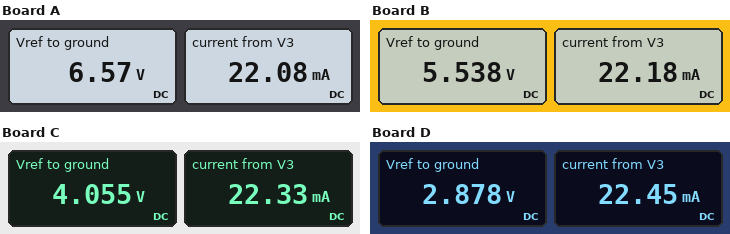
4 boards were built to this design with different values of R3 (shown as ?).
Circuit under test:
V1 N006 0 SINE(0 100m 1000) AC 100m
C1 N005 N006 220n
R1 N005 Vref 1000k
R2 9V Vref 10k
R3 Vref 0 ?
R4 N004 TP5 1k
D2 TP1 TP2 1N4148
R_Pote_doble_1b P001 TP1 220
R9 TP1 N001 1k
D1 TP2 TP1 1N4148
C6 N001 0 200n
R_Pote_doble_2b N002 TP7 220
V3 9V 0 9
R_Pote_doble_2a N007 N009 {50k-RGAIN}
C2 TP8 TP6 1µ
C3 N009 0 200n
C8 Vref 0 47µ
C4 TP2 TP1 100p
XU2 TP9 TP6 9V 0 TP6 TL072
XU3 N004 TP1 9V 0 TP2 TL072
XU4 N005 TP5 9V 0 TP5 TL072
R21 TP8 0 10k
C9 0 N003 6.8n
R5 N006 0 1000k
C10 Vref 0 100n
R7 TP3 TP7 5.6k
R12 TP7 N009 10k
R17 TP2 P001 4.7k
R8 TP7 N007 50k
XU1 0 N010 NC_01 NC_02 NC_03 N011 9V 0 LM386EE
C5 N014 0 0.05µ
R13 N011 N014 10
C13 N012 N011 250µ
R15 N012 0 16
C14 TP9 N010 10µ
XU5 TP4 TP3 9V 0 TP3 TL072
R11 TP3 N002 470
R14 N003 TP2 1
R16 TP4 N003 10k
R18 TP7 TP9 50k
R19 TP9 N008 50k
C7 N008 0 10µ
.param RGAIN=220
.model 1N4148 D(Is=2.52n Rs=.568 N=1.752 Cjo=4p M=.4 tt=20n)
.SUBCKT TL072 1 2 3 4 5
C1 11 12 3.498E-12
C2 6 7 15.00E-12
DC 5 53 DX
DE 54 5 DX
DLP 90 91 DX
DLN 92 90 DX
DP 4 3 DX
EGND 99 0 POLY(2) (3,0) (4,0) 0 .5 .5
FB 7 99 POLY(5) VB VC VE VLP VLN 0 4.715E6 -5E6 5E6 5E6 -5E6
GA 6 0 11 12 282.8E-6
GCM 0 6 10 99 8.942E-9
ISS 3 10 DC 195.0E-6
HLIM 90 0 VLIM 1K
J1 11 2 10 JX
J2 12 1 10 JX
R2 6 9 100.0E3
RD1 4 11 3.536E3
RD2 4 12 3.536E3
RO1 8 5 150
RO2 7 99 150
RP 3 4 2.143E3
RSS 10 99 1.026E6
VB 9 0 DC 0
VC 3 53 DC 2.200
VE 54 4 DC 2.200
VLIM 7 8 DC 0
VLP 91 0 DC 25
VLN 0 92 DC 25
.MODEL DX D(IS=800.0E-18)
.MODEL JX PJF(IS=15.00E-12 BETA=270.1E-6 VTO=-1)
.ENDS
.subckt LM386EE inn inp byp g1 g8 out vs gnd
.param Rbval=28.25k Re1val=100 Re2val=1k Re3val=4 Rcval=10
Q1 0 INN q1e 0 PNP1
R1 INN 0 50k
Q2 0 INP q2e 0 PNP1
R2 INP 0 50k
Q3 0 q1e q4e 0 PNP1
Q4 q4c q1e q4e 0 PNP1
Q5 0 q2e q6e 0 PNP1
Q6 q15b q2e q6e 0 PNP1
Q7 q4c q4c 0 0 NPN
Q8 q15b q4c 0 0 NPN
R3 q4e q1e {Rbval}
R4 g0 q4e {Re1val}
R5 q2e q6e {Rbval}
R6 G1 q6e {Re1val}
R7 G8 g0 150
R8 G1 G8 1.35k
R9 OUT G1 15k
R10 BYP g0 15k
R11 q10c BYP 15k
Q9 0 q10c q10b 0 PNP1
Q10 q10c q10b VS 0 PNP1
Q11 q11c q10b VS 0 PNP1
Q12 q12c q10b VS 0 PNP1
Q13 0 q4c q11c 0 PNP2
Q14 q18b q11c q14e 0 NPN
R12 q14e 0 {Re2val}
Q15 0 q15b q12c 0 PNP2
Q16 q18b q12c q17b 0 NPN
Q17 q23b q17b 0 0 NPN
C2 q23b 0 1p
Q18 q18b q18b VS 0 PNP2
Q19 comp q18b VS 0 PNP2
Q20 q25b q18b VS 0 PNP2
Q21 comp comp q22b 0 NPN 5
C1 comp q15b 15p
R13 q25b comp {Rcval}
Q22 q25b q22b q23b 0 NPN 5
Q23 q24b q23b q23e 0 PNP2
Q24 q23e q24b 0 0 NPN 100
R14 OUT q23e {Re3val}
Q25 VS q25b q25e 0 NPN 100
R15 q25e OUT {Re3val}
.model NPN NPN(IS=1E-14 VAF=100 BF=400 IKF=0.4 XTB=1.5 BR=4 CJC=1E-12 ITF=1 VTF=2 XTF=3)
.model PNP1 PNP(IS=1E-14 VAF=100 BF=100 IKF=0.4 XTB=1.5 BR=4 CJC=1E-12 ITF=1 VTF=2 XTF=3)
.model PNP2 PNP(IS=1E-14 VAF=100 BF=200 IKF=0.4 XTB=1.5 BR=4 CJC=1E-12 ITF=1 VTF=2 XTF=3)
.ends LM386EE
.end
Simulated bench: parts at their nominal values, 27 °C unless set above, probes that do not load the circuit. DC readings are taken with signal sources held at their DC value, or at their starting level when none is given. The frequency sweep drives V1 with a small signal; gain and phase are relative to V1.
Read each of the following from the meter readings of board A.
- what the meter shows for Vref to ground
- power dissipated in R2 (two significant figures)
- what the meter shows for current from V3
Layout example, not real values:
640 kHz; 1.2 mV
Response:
6.57 V; 590 µW; 22.08 mA
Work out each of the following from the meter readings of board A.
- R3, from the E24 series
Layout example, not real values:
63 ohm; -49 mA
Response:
27 kΩ
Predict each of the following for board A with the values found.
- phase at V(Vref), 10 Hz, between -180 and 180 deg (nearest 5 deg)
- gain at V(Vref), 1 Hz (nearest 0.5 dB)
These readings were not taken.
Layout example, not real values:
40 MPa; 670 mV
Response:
-85 deg; -52.0 dB
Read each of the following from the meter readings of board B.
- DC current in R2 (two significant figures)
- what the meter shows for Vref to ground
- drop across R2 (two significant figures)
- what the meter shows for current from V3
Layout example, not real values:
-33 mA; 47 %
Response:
350 µA; 5.538 V; 3.5 V; 22.18 mA
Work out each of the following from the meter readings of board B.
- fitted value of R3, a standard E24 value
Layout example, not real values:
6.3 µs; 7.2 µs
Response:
16 kΩ
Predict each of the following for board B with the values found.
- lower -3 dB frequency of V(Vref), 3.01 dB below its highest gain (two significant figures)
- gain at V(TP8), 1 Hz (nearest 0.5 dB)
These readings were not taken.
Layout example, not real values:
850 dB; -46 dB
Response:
260 mHz; -35.0 dB
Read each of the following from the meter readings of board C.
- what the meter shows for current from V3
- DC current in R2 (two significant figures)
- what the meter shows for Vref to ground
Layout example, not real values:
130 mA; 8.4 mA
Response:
22.33 mA; 490 µA; 4.055 V
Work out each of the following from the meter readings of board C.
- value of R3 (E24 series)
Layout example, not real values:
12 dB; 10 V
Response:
8.2 kΩ
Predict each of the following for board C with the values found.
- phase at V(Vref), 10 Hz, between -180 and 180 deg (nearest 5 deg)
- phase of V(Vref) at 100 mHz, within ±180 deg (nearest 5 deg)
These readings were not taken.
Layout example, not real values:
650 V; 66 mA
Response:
-80 deg; 75 deg
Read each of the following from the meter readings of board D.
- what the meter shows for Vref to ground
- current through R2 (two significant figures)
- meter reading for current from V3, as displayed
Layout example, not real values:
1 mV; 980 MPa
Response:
2.878 V; 610 µA; 22.45 mA
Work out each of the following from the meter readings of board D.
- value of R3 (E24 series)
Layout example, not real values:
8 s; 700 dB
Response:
4.7 kΩ
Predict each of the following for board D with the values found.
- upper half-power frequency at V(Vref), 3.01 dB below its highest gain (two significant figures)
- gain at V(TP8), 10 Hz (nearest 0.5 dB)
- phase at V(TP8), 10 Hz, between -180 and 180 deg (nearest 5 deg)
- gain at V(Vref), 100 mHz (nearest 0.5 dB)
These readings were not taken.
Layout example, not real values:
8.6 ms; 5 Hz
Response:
2.1 Hz; -15.0 dB; 65 deg; -67.0 dB
